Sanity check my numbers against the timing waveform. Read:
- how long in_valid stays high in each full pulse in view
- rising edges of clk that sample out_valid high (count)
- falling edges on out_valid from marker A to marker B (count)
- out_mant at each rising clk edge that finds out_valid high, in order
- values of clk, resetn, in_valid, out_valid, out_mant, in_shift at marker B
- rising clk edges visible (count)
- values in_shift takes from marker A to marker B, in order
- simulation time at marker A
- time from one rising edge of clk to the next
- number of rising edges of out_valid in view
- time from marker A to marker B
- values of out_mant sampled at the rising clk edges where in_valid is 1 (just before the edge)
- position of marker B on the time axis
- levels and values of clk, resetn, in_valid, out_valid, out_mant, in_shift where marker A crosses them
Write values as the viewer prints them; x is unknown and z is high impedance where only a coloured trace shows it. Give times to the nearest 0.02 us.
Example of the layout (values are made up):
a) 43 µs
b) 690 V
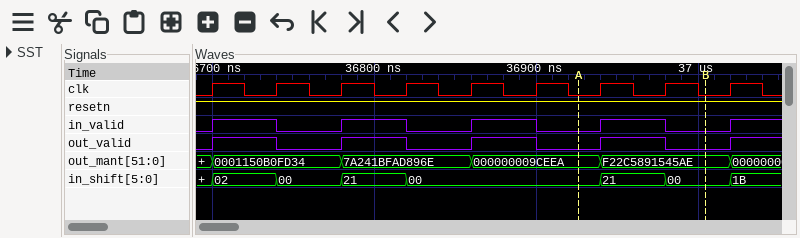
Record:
a) 0.04 us, 0.04 us, 0.04 us, 0.04 us
b) 4
c) 1
d) 0001150B0FD34, 7A241BFAD896E, 000000009CEEA, F22C5891545AE
e) clk=0, resetn=1, in_valid=0, out_valid=0, out_mant=F22C5891545AE, in_shift=00
f) 9
g) 00, 21, 00
h) 36.92 us
i) 0.04 us
j) 5
k) 0.08 us
l) 0001150B0FD34, 7A241BFAD896E, 000000009CEEA, F22C5891545AE
m) 37 us
n) clk=0, resetn=1, in_valid=0, out_valid=0, out_mant=000000009CEEA, in_shift=00
